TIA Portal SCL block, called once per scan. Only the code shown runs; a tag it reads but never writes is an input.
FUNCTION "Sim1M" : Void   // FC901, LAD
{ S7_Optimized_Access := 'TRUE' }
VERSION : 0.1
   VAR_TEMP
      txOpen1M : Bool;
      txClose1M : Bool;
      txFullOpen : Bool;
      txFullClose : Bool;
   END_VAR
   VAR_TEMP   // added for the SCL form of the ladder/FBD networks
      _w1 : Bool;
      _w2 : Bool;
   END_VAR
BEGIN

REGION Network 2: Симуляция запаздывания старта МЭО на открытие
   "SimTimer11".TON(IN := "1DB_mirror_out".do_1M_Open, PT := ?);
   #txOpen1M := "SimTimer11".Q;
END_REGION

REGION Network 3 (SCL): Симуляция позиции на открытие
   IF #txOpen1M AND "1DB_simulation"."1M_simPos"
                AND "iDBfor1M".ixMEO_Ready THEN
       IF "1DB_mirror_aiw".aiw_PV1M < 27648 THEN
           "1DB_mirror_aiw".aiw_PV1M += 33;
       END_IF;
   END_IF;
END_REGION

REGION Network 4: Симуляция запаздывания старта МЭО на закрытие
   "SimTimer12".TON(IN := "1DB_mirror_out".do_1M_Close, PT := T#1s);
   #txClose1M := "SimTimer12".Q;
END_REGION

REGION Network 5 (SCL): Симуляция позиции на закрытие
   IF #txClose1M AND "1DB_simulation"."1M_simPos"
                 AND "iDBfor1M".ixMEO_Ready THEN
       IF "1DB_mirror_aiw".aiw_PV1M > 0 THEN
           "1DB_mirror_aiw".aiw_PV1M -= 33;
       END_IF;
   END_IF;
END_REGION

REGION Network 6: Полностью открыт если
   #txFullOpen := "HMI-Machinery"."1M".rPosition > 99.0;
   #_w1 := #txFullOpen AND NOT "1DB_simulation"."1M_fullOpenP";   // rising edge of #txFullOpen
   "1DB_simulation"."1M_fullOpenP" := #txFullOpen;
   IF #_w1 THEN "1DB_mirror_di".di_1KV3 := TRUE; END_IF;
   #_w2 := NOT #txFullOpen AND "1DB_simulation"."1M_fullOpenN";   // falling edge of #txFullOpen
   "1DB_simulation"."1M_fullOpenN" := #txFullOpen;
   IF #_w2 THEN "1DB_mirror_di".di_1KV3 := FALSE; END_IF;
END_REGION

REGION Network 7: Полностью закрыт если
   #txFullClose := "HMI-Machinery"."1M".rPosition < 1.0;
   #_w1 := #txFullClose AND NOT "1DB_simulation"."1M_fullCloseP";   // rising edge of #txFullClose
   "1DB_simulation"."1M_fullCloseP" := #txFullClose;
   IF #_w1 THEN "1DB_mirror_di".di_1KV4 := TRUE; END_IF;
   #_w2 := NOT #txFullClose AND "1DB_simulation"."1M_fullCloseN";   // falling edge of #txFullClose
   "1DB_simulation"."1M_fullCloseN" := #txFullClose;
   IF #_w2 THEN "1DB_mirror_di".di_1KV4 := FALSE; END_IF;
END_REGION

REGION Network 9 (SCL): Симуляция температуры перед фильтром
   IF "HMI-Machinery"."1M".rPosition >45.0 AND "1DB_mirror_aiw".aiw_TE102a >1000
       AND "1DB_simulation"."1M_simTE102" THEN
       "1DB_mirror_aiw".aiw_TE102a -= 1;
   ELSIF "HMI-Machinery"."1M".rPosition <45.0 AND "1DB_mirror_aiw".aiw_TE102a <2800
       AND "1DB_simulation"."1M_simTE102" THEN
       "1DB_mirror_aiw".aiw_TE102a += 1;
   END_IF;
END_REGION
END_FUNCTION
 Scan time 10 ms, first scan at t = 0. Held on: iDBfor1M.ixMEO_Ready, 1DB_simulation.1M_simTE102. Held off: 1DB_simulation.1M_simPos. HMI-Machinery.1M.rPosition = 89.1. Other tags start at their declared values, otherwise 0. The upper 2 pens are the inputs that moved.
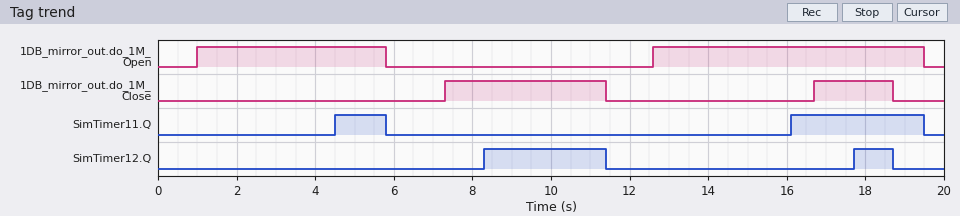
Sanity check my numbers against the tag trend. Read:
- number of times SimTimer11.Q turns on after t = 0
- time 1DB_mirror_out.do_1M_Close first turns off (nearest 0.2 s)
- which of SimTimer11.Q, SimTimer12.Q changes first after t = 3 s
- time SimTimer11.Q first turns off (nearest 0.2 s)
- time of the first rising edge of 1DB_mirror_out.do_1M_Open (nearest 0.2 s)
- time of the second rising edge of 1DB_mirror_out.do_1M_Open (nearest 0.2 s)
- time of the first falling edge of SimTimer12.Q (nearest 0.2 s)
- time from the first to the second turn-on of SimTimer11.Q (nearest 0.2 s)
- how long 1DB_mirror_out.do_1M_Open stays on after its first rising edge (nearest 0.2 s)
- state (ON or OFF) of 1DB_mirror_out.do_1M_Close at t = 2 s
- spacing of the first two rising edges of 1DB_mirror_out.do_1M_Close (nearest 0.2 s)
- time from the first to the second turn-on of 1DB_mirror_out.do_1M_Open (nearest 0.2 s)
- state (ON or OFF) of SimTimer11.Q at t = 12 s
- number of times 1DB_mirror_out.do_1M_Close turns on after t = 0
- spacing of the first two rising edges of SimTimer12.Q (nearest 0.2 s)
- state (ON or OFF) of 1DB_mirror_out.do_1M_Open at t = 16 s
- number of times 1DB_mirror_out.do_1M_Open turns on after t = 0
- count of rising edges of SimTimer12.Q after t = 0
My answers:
2
11.4 s
SimTimer11.Q
5.8 s
1.0 s
12.6 s
11.4 s
11.6 s
4.8 s
OFF
9.4 s
11.6 s
OFF
2
9.4 s
ON
2
2
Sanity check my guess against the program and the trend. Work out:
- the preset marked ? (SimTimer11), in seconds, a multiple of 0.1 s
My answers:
3.5 s
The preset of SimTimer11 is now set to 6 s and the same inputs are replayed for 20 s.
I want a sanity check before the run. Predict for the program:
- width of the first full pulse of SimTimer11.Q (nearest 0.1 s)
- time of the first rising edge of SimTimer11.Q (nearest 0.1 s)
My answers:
0.9 s
18.6 s
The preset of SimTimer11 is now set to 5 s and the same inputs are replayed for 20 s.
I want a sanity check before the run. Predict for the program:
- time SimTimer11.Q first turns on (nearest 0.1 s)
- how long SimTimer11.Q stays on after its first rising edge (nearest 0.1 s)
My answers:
17.6 s
1.9 s
